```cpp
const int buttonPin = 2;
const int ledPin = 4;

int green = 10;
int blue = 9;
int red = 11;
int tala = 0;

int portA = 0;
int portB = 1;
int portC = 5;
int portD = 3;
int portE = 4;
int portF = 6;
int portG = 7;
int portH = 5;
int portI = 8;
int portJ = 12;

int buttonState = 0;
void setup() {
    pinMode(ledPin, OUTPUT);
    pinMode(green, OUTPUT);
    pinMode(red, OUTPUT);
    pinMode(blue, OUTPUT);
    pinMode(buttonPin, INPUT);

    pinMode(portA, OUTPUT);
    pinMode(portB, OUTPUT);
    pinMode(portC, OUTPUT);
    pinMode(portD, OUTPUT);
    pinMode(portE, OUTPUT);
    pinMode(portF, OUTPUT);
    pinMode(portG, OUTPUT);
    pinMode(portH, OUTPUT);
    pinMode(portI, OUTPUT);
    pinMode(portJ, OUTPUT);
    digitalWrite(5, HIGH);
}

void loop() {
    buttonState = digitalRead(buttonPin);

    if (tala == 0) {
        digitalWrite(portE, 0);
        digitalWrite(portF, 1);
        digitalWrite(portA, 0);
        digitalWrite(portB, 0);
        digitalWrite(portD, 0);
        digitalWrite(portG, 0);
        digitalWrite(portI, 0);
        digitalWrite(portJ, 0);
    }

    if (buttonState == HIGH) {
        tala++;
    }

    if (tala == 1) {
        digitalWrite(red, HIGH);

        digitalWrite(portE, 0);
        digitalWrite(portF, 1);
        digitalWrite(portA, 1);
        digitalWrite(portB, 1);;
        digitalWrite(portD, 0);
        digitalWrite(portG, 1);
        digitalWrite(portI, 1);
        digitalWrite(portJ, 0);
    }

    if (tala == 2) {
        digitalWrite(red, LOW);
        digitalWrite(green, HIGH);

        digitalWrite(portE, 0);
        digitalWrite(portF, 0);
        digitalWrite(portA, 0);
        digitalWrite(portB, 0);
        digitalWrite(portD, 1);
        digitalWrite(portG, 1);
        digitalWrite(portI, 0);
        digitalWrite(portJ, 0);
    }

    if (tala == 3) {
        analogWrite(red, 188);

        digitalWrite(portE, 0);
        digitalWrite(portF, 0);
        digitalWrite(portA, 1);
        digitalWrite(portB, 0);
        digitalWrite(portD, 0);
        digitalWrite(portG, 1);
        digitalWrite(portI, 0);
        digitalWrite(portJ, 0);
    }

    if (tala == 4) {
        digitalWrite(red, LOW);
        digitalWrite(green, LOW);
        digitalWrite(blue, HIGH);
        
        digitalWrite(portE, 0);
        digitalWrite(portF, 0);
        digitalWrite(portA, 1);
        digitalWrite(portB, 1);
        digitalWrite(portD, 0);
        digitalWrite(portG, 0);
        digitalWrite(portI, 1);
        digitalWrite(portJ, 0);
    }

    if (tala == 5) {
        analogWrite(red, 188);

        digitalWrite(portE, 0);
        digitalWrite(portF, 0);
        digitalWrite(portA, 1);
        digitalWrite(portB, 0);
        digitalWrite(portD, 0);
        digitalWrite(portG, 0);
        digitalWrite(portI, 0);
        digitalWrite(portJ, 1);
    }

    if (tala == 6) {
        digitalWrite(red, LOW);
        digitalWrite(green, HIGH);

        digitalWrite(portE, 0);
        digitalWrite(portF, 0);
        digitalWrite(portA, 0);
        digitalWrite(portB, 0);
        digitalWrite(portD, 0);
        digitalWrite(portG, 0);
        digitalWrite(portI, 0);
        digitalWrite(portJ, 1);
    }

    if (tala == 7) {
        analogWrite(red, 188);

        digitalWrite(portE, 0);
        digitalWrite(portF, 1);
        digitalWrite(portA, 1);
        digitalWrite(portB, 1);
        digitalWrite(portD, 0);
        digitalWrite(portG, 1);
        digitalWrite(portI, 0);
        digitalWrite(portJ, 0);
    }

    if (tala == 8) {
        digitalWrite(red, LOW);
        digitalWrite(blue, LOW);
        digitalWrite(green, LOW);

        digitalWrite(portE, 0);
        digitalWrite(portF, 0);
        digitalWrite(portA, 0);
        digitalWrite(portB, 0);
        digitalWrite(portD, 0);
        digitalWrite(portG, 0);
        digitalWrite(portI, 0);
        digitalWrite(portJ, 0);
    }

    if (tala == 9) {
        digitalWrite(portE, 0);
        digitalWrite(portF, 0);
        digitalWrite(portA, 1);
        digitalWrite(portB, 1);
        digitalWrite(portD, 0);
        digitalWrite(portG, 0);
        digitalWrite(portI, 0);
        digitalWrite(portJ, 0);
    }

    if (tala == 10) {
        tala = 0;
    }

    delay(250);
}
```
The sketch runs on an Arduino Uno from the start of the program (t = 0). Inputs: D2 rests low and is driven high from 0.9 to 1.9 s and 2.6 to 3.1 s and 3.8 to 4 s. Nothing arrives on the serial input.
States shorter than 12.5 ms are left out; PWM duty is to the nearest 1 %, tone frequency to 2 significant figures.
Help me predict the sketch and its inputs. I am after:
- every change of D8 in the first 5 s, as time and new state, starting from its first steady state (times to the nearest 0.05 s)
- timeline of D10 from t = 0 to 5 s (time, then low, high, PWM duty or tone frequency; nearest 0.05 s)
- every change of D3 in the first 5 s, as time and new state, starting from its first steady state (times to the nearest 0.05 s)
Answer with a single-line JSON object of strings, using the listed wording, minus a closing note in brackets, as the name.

{"every change of D8 in the first 5 s, as time and new state, starting from its first steady state": "0 s low; 1 s high; 1.25 s low; 1.75 s high; 2.75 s low", "timeline of D10 from t = 0 to 5 s": "0 s low; 1.25 s high; 1.75 s low; 3 s high", "every change of D3 in the first 5 s, as time and new state, starting from its first steady state": "0 s low; 1.25 s high; 1.5 s low"}
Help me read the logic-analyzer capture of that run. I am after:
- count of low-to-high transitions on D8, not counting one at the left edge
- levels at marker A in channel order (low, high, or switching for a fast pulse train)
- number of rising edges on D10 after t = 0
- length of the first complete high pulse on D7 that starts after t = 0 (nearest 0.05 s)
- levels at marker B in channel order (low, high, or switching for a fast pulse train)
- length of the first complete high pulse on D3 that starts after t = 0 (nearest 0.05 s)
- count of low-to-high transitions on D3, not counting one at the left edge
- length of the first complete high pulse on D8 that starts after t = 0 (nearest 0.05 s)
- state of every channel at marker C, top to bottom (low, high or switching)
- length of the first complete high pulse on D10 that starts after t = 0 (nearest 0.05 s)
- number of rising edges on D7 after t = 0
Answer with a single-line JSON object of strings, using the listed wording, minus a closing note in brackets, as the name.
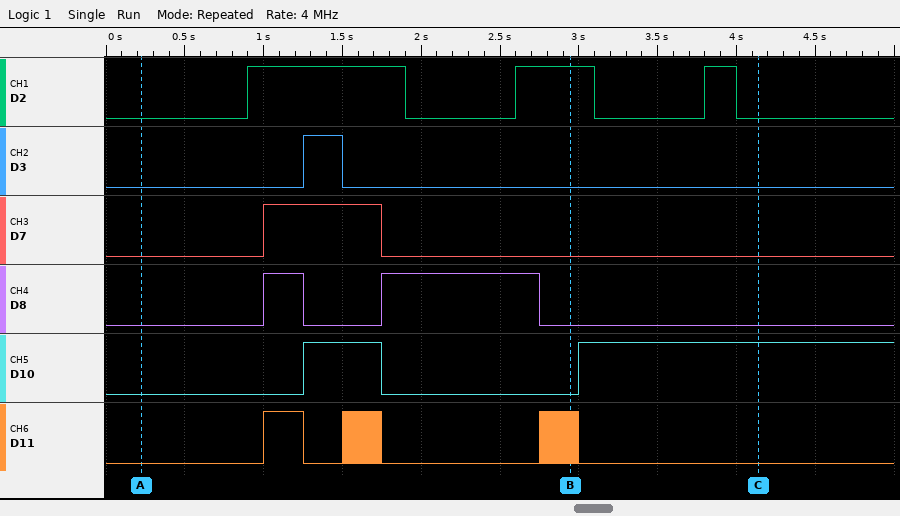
{"count of low-to-high transitions on D8, not counting one at the left edge": "2", "levels at marker A in channel order": "D2 low, D3 low, D7 low, D8 low, D10 low, D11 low", "number of rising edges on D10 after t = 0": "2", "length of the first complete high pulse on D7 that starts after t = 0": "0.75 s", "levels at marker B in channel order": "D2 high, D3 low, D7 low, D8 low, D10 low, D11 switching", "length of the first complete high pulse on D3 that starts after t = 0": "0.25 s", "count of low-to-high transitions on D3, not counting one at the left edge": "1", "length of the first complete high pulse on D8 that starts after t = 0": "0.25 s", "state of every channel at marker C, top to bottom": "D2 low, D3 low, D7 low, D8 low, D10 high, D11 low", "length of the first complete high pulse on D10 that starts after t = 0": "0.50 s", "number of rising edges on D7 after t = 0": "1"}
